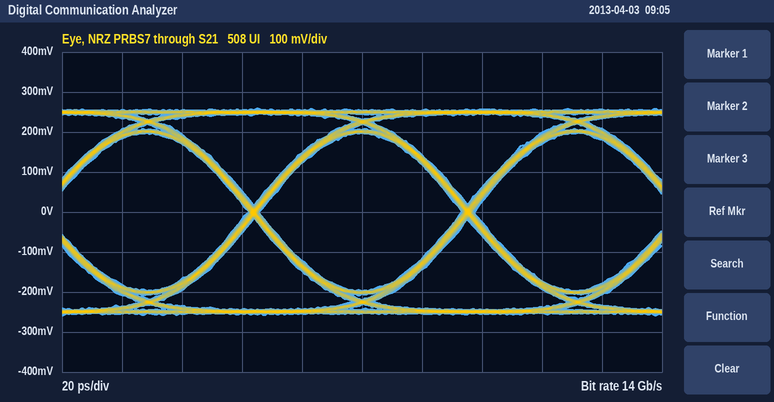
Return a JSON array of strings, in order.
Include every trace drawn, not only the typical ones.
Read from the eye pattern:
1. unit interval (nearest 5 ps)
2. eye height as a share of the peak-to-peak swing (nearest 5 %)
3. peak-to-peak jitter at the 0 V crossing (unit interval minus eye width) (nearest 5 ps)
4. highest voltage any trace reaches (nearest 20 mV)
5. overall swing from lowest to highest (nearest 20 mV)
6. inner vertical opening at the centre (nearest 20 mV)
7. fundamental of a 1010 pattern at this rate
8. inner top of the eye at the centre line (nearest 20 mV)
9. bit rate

["70 ps", "75 %", "5 ps", "260 mV", "520 mV", "400 mV", "7 GHz", "200 mV", "14 Gb/s"]
